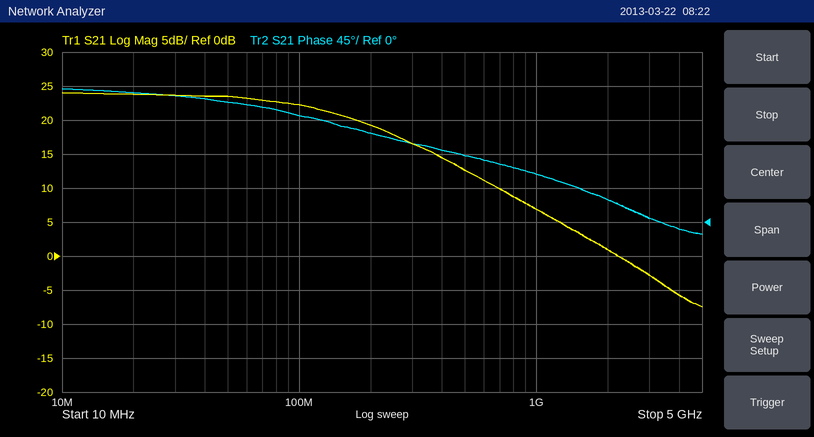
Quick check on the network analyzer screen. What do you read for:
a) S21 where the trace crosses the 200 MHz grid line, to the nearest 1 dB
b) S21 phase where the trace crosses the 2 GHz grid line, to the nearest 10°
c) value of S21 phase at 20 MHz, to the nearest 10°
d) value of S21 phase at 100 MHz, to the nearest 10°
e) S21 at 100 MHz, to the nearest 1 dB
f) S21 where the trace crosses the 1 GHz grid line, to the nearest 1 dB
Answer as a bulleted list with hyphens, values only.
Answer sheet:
- 19 dB
- 30°
- 170°
- 140°
- 22 dB
- 7 dB
